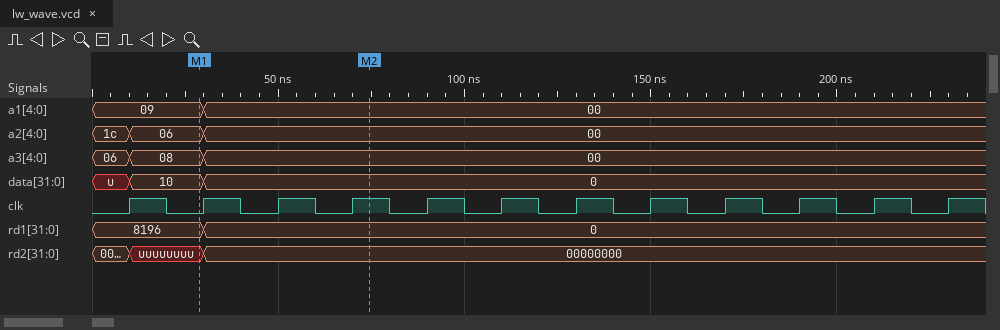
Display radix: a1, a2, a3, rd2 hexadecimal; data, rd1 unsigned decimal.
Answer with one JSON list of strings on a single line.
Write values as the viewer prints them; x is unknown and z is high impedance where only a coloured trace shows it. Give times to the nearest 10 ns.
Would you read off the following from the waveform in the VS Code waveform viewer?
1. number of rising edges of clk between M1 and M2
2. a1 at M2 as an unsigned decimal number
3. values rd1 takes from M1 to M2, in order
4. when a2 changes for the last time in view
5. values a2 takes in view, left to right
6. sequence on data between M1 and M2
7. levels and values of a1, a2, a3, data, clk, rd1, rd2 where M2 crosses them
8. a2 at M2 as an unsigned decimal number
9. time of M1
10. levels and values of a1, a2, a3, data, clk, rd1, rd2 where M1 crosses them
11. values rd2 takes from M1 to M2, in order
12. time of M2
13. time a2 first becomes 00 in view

["3", "0", "8196, 0", "30 ns", "1c, 06, 00", "10, 0", "a1=00, a2=00, a3=00, data=0, clk=1, rd1=0, rd2=00000000", "0", "30 ns", "a1=09, a2=06, a3=08, data=10, clk=0, rd1=8196, rd2=uuuuuuuu", "uuuuuuuu, 00000000", "70 ns", "30 ns"]
